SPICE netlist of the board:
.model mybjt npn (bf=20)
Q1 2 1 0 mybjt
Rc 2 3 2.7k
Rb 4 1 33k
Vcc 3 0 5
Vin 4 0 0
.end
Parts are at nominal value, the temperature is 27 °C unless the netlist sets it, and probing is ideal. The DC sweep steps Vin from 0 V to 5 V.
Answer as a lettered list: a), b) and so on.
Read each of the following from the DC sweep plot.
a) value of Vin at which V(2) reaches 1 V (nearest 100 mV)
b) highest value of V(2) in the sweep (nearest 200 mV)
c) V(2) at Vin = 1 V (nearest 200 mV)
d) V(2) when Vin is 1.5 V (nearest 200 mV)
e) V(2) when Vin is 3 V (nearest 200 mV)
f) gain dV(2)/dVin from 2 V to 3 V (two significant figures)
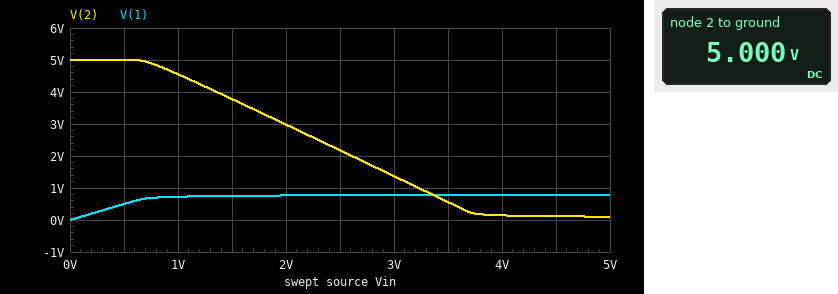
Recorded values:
a) 3.2 V
b) 5.0 V
c) 4.6 V
d) 3.8 V
e) 1.4 V
f) -1.6 V/V
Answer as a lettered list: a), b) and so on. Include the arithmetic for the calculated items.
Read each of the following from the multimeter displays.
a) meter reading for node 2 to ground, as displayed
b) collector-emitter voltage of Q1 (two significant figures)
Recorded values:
a) 5.000 V
b) 5 V = 5.0 V
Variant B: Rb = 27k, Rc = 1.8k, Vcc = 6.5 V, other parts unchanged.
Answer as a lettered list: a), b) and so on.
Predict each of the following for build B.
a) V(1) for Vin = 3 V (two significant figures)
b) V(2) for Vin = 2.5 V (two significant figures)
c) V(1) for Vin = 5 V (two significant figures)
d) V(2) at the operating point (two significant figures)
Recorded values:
a) 790 mV
b) 4.2 V
c) 800 mV
d) 6.5 V
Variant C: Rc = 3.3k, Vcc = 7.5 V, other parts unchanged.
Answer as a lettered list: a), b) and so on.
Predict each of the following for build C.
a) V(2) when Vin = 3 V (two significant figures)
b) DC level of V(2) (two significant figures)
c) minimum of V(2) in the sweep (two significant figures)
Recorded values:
a) 3.1 V
b) 7.5 V
c) 130 mV
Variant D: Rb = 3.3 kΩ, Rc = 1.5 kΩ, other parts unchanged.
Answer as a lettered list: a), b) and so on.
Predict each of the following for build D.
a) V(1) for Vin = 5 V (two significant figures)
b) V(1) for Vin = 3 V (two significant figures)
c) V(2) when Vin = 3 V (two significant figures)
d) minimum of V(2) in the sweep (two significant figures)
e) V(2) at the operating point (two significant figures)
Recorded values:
a) 820 mV
b) 810 mV
c) 58 mV
d) 43 mV
e) 5.0 V
